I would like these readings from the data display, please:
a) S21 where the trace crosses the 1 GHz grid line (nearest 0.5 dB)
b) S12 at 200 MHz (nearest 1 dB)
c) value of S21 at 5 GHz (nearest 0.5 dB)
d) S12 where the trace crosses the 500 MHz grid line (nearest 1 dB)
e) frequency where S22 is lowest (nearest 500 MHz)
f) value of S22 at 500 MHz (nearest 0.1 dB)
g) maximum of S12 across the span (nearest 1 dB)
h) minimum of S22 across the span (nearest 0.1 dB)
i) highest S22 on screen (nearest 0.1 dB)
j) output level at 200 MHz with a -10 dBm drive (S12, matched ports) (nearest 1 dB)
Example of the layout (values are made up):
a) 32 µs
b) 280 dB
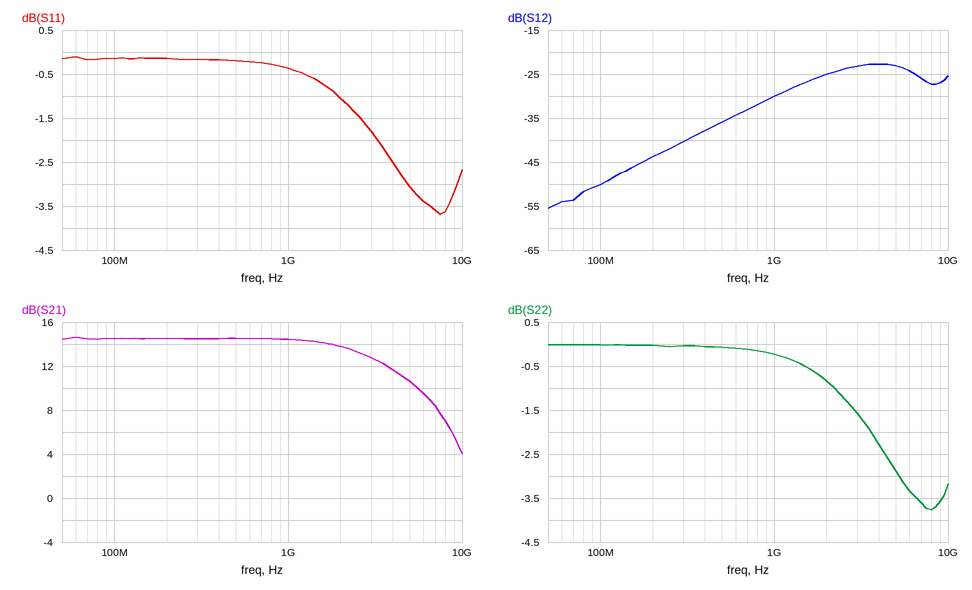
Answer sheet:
a) 14.5 dB
b) -44 dB
c) 10.5 dB
d) -36 dB
e) 8.0 GHz
f) -0.1 dB
g) -23 dB
h) -3.8 dB
i) 0.0 dB
j) -54 dBm
